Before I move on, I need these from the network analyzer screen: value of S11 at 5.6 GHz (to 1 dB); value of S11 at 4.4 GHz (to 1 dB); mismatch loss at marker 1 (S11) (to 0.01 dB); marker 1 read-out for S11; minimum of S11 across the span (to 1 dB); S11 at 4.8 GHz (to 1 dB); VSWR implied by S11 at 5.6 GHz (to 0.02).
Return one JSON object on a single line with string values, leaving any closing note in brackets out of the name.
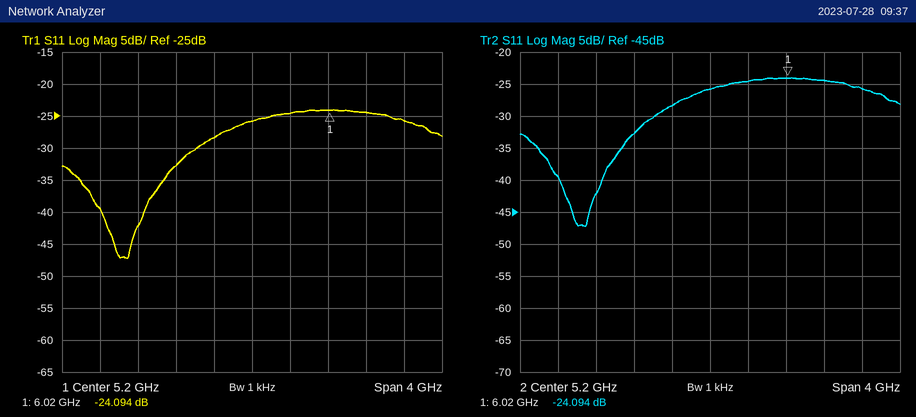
{"value of S11 at 5.6 GHz": "-25 dB", "value of S11 at 4.4 GHz": "-33 dB", "mismatch loss at marker 1 (S11)": "0.02 dB", "marker 1 read-out for S11": "-24.094 dB", "minimum of S11 across the span": "-47 dB", "S11 at 4.8 GHz": "-28 dB", "VSWR implied by S11 at 5.6 GHz": "1.12"}
